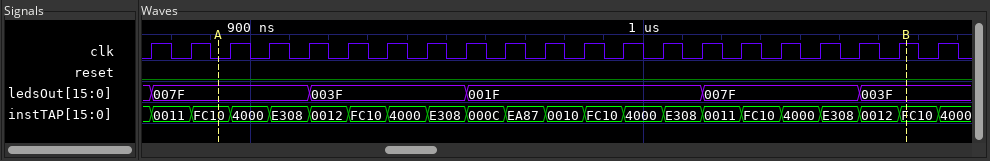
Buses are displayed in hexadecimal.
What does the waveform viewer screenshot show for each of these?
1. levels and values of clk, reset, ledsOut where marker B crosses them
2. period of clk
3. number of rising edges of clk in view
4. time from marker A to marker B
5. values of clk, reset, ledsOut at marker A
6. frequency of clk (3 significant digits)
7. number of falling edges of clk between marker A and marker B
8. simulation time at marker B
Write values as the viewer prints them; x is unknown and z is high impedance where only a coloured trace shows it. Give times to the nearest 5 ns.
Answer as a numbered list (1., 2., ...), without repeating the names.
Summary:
1. clk=1, reset=0, ledsOut=003F
2. 10 ns
3. 21
4. 175 ns
5. clk=0, reset=0, ledsOut=007F
6. 100 MHz
7. 17
8. 1065 ns
